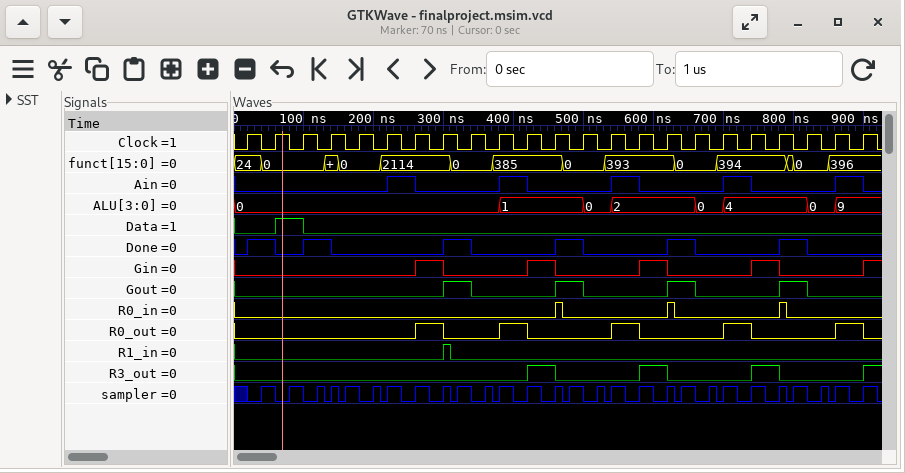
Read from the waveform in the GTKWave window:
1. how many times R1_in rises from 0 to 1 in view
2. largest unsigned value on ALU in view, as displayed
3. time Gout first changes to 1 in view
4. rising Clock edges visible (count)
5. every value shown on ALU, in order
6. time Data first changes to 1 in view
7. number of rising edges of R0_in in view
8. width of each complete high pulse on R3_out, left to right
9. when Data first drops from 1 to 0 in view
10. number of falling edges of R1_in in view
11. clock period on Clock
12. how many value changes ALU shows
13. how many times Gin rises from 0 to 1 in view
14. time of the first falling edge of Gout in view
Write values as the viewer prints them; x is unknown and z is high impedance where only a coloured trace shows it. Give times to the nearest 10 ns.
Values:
1
9
300 ns
23
0, 1, 0, 2, 0, 4, 0, 9
60 ns
3
40 ns, 40 ns, 40 ns
100 ns
1
40 ns
7
5
340 ns
